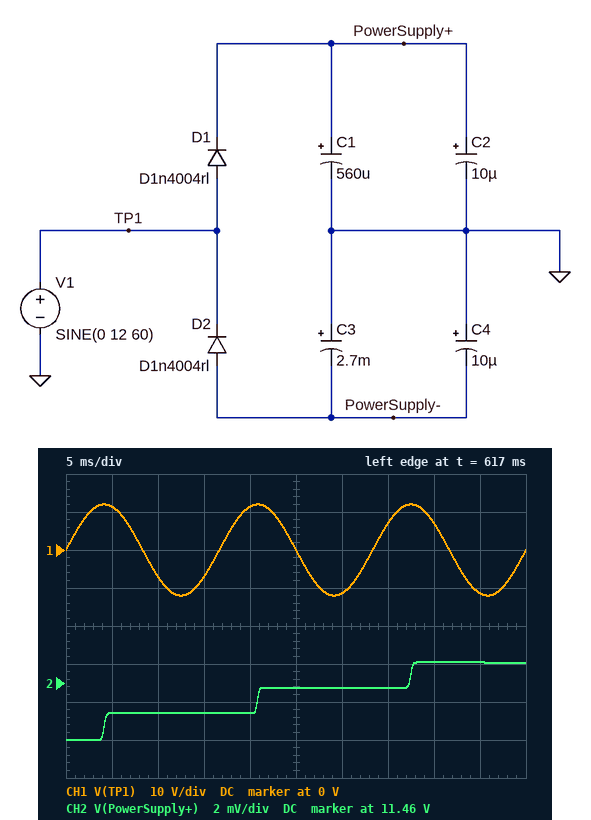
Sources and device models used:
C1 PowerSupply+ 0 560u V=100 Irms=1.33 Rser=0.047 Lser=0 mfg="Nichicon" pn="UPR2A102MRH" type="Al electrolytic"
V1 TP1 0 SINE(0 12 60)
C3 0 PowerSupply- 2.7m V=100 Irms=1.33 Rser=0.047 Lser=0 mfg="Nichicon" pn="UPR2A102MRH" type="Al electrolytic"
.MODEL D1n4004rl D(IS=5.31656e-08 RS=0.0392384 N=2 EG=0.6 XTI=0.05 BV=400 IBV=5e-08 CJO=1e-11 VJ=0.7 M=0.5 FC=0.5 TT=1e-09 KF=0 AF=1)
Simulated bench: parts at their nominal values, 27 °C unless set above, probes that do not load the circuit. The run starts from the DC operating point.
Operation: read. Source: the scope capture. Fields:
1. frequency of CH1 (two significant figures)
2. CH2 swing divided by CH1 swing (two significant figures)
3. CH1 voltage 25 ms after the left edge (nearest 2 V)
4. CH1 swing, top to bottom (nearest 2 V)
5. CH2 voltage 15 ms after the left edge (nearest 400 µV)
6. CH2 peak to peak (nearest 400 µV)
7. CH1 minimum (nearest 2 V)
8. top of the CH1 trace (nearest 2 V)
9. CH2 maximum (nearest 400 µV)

60 Hz
0.00017
0 V
24 V
11.4604 V
4.0 mV
-12 V
12 V
11.4632 V
